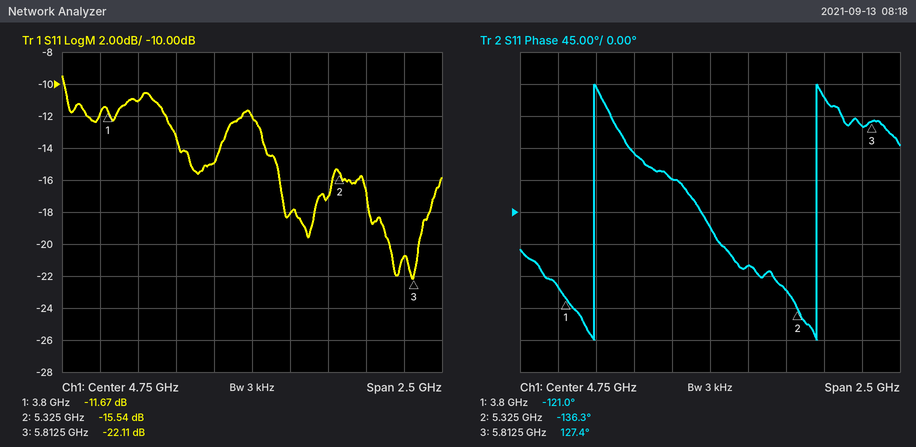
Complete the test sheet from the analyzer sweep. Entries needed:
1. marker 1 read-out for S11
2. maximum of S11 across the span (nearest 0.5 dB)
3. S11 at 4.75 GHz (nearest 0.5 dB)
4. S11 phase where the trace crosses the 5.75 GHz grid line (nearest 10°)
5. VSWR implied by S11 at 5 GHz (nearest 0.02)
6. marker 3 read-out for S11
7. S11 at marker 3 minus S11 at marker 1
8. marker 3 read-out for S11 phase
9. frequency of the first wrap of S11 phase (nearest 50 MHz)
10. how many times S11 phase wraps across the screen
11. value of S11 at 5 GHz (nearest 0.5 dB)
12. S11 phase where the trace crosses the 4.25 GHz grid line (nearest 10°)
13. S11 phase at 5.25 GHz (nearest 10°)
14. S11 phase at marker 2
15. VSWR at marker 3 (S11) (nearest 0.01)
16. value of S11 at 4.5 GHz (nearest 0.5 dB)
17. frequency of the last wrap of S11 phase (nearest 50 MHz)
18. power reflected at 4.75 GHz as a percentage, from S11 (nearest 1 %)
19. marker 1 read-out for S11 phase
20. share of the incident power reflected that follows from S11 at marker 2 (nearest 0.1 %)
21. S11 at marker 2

-11.67 dB
-9.5 dB
-12.0 dB
120°
1.28
-22.11 dB
-10.44 dB
127.4°
4.00 GHz
2
-18.0 dB
80°
-110°
-136.3°
1.17
-15.0 dB
5.45 GHz
6 %
-121.0°
2.8 %
-15.54 dB
